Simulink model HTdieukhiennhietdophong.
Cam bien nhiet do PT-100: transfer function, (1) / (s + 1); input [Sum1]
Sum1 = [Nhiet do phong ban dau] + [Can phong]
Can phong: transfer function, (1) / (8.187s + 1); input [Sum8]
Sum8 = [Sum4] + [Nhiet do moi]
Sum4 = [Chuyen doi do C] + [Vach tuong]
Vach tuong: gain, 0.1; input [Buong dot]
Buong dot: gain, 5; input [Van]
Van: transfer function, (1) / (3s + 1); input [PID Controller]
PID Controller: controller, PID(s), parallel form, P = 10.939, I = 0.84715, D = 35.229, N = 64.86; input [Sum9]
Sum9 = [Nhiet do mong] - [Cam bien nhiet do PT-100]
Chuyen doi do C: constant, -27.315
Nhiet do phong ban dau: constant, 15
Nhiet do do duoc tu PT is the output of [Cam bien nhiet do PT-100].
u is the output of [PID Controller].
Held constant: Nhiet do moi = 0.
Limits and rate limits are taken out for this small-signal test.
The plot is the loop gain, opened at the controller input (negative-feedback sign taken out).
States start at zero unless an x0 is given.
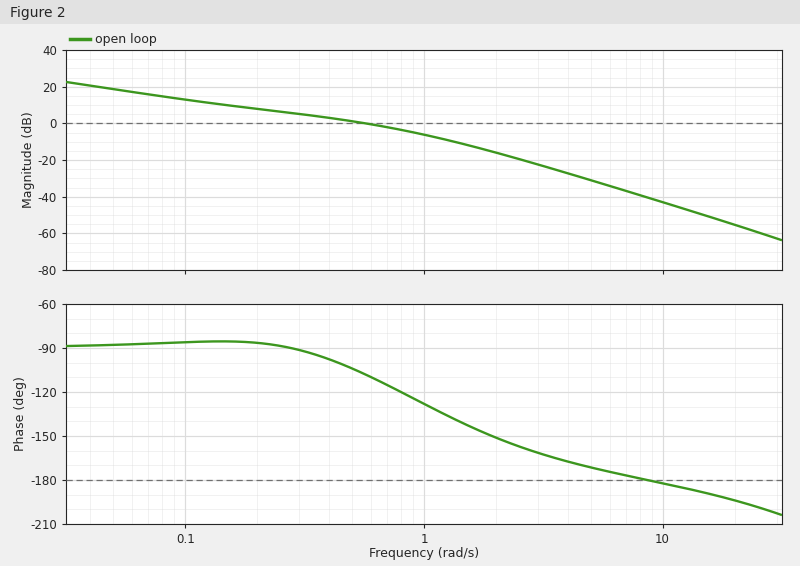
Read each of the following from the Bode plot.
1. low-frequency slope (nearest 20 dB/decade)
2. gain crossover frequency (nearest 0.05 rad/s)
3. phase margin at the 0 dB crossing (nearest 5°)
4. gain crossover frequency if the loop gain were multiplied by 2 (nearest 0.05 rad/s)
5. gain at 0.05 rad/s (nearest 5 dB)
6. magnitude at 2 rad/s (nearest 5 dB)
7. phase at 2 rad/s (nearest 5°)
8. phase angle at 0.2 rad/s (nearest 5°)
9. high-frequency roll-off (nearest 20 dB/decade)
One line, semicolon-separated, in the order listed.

-20 dB/decade; 0.55 rad/s; 70°; 1.00 rad/s; 20 dB; -15 dB; -150°; -85°; -40 dB/decade
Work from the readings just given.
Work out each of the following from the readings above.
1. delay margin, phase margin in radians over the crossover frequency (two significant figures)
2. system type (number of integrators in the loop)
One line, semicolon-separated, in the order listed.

2.2 s; 1
